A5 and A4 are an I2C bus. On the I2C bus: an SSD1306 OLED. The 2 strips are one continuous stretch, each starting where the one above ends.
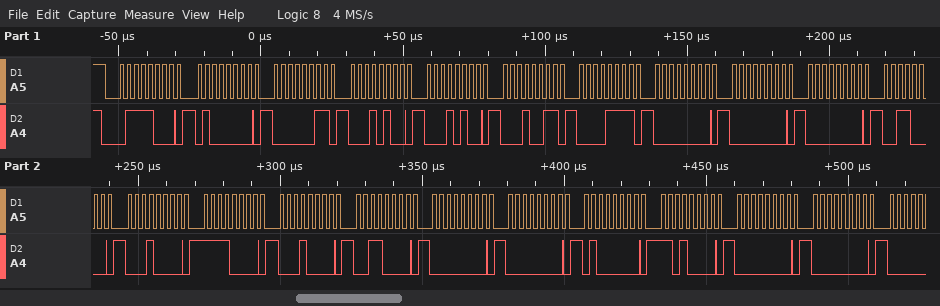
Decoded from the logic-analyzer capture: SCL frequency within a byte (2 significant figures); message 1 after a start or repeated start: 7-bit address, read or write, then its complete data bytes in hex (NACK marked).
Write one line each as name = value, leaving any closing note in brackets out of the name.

SCL frequency within a byte = 400 kHz
message 1 after a start or repeated start: 7-bit address, read or write, then its complete data bytes in hex = 0x3C write: 40 03 14 14 13 0F 00 00 00 30 10 F0 10 30 00 00 40 D0 00 00
